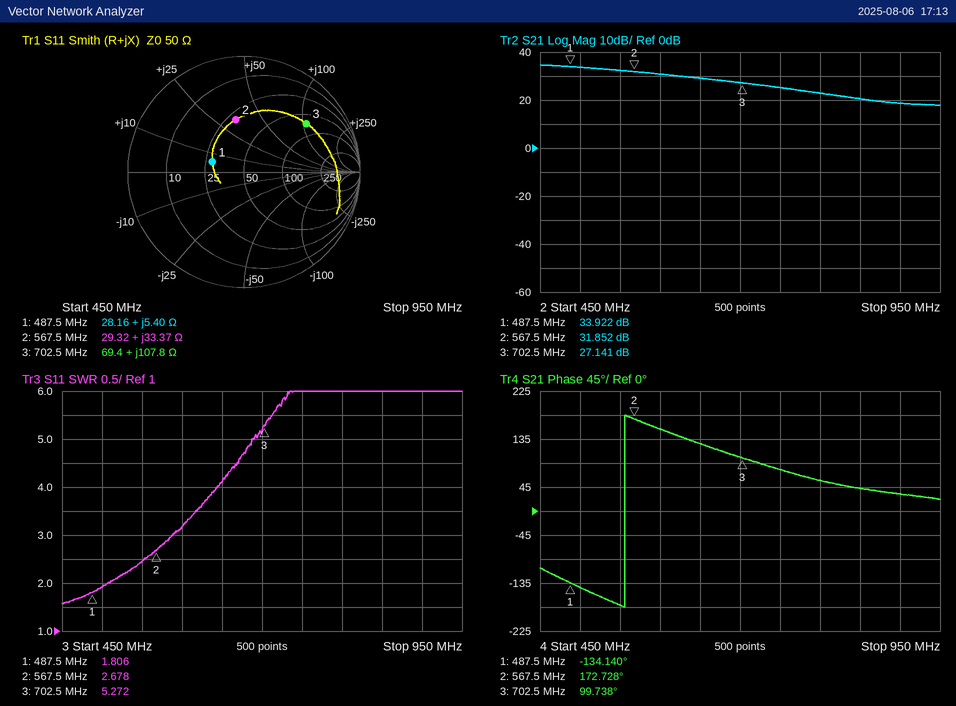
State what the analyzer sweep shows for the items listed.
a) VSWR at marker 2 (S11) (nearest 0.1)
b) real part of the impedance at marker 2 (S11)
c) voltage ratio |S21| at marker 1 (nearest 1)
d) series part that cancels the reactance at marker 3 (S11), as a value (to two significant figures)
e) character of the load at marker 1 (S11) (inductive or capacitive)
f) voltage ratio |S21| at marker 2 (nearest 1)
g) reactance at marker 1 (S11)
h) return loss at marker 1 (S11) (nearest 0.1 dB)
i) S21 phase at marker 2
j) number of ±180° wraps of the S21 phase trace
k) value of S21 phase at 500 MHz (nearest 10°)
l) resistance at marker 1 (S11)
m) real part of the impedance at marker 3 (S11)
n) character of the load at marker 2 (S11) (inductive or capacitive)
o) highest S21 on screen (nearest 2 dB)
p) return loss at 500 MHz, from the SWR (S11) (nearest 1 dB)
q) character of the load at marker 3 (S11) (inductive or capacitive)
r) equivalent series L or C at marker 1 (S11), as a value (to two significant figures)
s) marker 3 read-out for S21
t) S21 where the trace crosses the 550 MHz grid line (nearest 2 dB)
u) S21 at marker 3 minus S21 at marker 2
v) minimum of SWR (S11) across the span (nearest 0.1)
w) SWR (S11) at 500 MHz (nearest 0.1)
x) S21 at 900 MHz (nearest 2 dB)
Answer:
2.7
29.32 Ω
50
2.1 pF
inductive
39
+5.40 Ω
10.8 dB
172.728°
1
-140°
28.16 Ω
69.4 Ω
inductive
34 dB
10 dB
inductive
1.8 nH
27.141 dB
32 dB
-4.711 dB
1.6
1.9
18 dB
